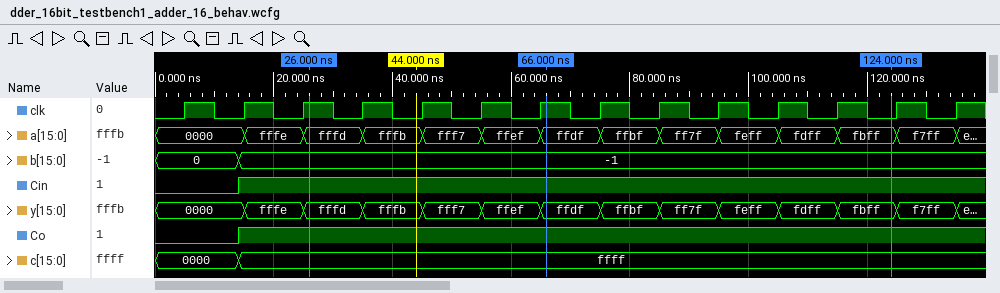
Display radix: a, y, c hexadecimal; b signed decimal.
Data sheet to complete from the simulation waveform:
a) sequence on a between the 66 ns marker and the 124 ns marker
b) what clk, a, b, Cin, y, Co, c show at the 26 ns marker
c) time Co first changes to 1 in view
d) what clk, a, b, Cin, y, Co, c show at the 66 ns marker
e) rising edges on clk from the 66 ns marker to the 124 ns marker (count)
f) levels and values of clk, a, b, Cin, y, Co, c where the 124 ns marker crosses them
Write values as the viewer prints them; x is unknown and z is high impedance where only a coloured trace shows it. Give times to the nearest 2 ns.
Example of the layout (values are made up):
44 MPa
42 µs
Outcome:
ffdf, ffbf, ff7f, feff, fdff, fbff
clk=1, a=fffd, b=-1, Cin=1, y=fffd, Co=1, c=ffff
14 ns
clk=1, a=ffdf, b=-1, Cin=1, y=ffdf, Co=1, c=ffff
5
clk=0, a=fbff, b=-1, Cin=1, y=fbff, Co=1, c=ffff
